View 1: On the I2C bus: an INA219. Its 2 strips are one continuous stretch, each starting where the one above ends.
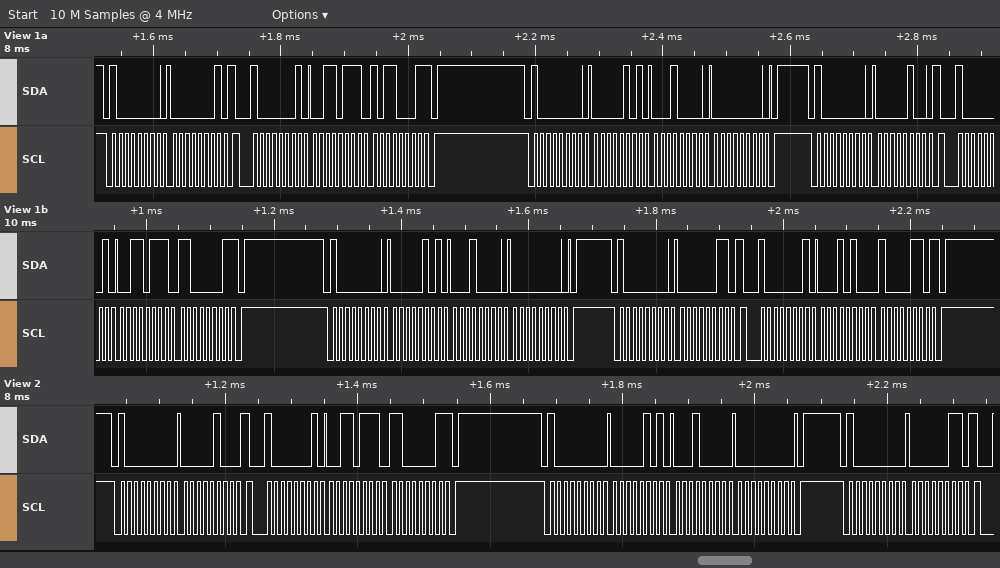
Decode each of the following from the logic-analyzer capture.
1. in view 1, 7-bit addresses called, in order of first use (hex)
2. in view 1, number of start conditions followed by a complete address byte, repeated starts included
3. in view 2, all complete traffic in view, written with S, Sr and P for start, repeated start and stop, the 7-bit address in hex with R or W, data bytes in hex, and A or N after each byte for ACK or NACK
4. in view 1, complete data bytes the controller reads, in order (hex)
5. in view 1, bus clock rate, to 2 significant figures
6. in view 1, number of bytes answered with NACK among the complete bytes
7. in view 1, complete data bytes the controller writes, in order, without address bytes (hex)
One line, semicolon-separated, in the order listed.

0x40; 8; S 40W A 04 A Sr 40R A 37 A C1 N P S 40W A 05 A 10 A 00 A P S 40W A 03 A; 37 B1 37 C1 14 86; 100 kHz; 3; 01 05 10 00 04 05 10 00 03
